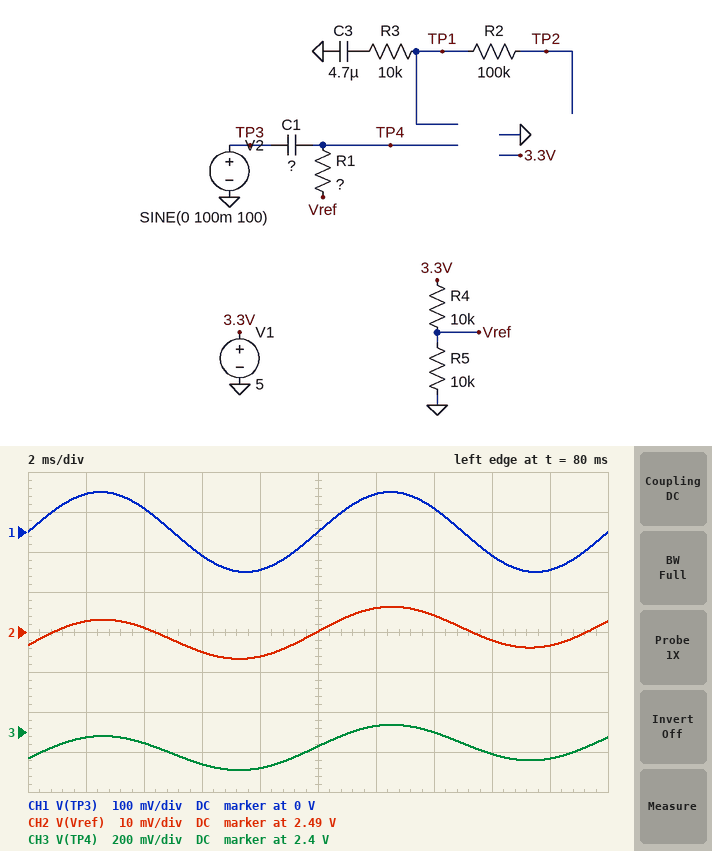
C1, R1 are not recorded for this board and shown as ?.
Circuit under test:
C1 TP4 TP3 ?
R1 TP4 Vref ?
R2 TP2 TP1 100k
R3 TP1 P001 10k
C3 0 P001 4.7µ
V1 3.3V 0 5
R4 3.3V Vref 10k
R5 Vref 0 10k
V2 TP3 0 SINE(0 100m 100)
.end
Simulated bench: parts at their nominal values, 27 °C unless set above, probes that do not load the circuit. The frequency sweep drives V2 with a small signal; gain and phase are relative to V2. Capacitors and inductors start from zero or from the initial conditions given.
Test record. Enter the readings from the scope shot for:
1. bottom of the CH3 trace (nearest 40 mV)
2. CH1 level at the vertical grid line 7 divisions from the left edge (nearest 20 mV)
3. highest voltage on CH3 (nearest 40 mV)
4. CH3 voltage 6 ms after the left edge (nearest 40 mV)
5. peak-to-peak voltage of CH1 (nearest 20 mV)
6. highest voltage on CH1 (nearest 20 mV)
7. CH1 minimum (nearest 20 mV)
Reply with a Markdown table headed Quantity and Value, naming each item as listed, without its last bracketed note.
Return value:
| Quantity | Value |
|---|---|
| bottom of the CH3 trace | 2.20 V |
| CH1 level at the vertical grid line 7 divisions from the left edge | 60 mV |
| highest voltage on CH3 | 2.44 V |
| CH3 voltage 6 ms after the left edge | 2.24 V |
| peak-to-peak voltage of CH1 | 200 mV |
| highest voltage on CH1 | 100 mV |
| CH1 minimum | -100 mV |
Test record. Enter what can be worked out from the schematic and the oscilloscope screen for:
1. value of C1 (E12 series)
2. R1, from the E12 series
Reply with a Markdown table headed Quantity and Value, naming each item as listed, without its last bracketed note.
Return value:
| Quantity | Value |
|---|---|
| value of C1 | 390 nF |
| R1, from the E12 series | 82 kΩ |
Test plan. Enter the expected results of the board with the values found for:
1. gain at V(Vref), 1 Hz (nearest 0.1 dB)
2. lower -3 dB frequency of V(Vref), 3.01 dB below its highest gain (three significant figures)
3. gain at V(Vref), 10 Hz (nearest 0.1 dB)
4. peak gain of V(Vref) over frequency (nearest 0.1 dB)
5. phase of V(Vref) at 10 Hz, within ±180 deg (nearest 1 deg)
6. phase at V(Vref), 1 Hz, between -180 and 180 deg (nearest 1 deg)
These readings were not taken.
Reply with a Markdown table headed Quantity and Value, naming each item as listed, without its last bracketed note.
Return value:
| Quantity | Value |
|---|---|
| gain at V(Vref), 1 Hz | -38.4 dB |
| lower -3 dB frequency of V(Vref), 3.01 dB below its highest gain | 4.69 Hz |
| gain at V(Vref), 10 Hz | -25.7 dB |
| peak gain of V(Vref) over frequency | -24.8 dB |
| phase of V(Vref) at 10 Hz, within ±180 deg | 25 deg |
| phase at V(Vref), 1 Hz, between -180 and 180 deg | 78 deg |
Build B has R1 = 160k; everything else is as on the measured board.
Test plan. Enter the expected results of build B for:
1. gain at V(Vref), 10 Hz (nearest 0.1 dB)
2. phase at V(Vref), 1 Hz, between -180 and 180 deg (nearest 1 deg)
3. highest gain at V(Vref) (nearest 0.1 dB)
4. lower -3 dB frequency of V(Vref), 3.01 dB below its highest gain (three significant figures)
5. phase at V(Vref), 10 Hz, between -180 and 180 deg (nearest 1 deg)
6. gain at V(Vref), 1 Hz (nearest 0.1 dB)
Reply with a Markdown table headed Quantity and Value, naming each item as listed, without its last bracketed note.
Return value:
| Quantity | Value |
|---|---|
| gain at V(Vref), 10 Hz | -30.6 dB |
| phase at V(Vref), 1 Hz, between -180 and 180 deg | 68 deg |
| highest gain at V(Vref) | -30.4 dB |
| lower -3 dB frequency of V(Vref), 3.01 dB below its highest gain | 2.47 Hz |
| phase at V(Vref), 10 Hz, between -180 and 180 deg | 14 deg |
| gain at V(Vref), 1 Hz | -38.9 dB |
